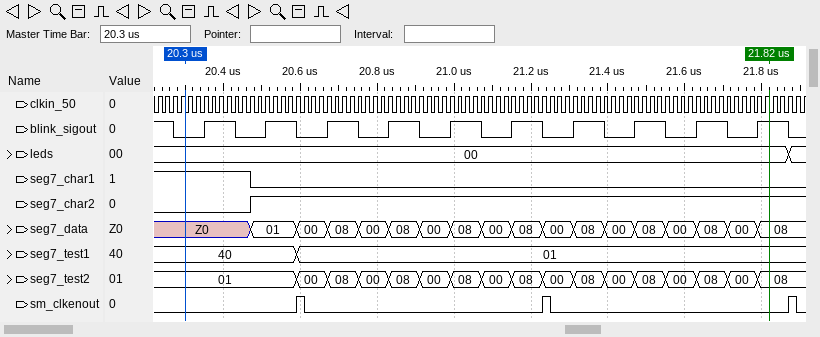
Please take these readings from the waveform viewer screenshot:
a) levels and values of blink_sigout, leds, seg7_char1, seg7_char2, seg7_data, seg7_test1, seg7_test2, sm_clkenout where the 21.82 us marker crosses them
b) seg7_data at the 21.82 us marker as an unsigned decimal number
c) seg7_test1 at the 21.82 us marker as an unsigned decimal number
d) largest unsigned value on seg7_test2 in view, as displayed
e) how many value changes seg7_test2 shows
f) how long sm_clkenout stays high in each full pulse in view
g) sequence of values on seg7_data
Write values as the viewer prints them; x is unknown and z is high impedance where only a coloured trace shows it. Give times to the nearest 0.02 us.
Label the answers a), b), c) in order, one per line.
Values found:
a) blink_sigout=1, leds=00, seg7_char1=0, seg7_char2=1, seg7_data=08, seg7_test1=01, seg7_test2=08, sm_clkenout=0
b) 8
c) 1
d) 08
e) 16
f) 0.02 us, 0.02 us, 0.02 us
g) Z0, 01, 00, 08, 00, 08, 00, 08, 00, 08, 00, 08, 00, 08, 00, 08, 00, 08
